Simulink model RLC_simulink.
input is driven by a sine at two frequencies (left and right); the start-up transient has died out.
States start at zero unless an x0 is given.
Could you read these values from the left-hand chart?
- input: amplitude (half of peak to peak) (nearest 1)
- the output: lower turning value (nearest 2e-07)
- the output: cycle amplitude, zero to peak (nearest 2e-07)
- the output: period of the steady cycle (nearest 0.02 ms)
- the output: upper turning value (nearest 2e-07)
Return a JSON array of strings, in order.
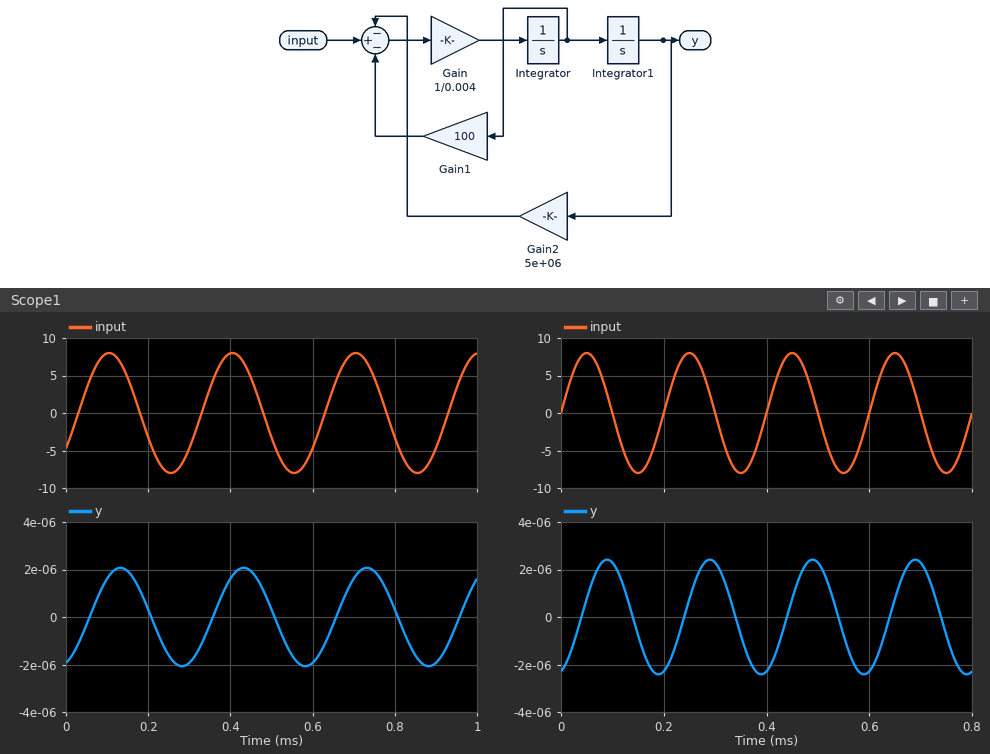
["8", "-0.0000020", "0.0000020", "0.30 ms", "0.0000020"]
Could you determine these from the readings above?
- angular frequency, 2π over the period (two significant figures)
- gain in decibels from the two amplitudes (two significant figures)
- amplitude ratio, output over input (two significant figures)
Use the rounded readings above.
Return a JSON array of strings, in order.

["21 rad/ms", "-130 dB", "0.00000025"]
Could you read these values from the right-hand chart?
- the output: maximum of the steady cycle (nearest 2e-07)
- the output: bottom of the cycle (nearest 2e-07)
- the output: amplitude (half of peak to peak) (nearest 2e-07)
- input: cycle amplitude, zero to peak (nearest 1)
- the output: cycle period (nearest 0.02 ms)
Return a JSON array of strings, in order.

["0.0000024", "-0.0000024", "0.0000024", "8", "0.20 ms"]
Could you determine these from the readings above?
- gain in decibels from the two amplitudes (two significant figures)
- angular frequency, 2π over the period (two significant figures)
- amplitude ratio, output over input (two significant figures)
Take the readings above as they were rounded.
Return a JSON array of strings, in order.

["-130 dB", "31 rad/ms", "0.00000030"]
